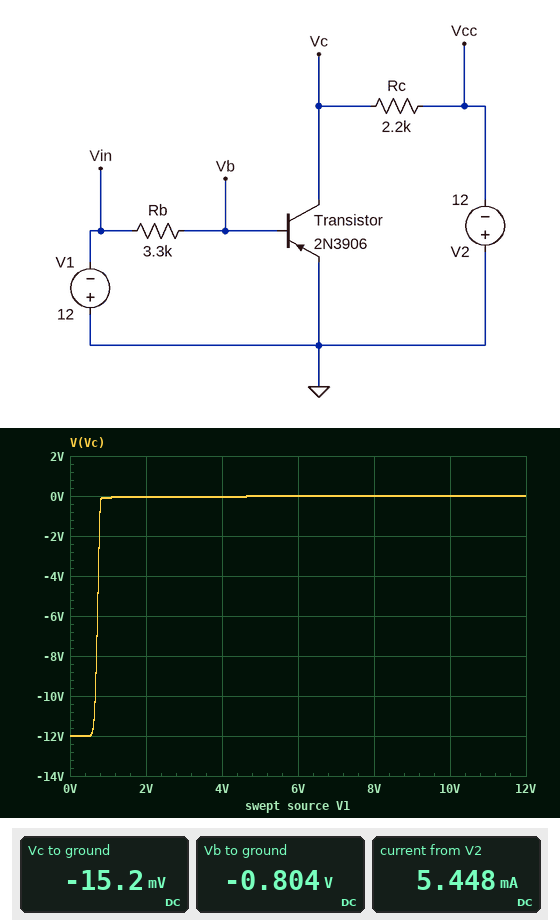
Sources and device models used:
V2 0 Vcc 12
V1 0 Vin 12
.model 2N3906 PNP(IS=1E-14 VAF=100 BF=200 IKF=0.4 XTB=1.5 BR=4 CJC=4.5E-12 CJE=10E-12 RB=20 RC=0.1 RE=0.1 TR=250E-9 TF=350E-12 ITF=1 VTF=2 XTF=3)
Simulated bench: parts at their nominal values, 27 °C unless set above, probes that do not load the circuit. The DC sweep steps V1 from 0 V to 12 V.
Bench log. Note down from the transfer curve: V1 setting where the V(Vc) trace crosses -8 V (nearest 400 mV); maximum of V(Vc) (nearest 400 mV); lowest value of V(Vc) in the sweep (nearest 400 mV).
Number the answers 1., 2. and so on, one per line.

1. 800 mV
2. 0 V
3. -12.0 V
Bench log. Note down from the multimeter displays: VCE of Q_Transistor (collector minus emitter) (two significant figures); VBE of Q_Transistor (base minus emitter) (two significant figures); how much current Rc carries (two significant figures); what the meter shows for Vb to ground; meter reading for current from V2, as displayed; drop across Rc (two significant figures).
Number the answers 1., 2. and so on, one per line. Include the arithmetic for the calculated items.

1. -15.2 mV = -15 mV
2. -804 mV = -800 mV
3. (-15.2 mV - (-12 V)) / 2.2 kΩ = 5.4 mA
4. -0.804 V
5. 5.448 mA
6. -15.2 mV - (-12 V) = 12 V
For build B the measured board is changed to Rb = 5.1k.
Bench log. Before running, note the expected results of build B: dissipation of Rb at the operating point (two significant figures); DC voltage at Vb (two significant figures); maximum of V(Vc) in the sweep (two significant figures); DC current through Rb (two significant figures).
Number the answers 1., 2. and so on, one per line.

1. 25 mW
2. -770 mV
3. -18 mV
4. 2.2 mA
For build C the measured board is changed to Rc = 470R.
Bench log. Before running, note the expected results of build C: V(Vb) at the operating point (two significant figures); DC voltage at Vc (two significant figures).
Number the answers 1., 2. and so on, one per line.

1. -820 mV
2. -38 mV
